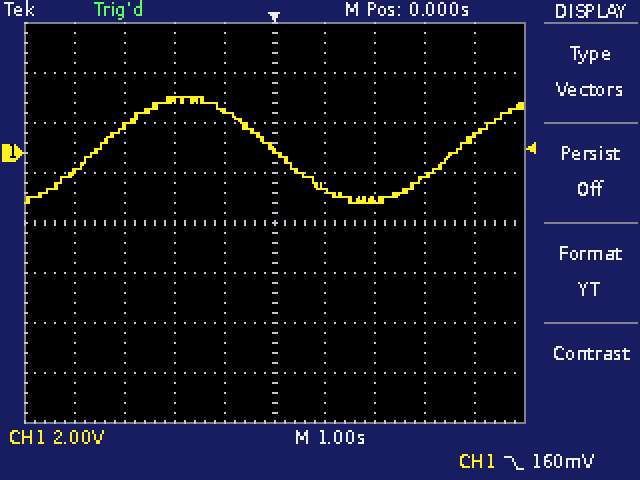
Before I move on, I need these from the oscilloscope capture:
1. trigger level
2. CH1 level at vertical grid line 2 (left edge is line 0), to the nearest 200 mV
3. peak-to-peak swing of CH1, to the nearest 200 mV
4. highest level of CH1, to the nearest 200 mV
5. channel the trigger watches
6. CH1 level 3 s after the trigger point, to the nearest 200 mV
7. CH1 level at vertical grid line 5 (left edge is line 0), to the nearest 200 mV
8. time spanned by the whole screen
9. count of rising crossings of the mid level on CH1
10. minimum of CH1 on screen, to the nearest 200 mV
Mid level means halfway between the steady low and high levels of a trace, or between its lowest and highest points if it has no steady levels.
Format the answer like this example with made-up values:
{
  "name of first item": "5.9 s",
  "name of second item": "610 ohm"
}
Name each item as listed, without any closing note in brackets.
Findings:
{
  "trigger level": "160 mV",
  "CH1 level at vertical grid line 2 (left edge is line 0), to the nearest 200 mV": "1.0 V",
  "peak-to-peak swing of CH1, to the nearest 200 mV": "4.2 V",
  "highest level of CH1, to the nearest 200 mV": "2.2 V",
  "channel the trigger watches": "CH1",
  "CH1 level 3 s after the trigger point, to the nearest 200 mV": "-1.0 V",
  "CH1 level at vertical grid line 5 (left edge is line 0), to the nearest 200 mV": "200 mV",
  "time spanned by the whole screen": "10 s",
  "count of rising crossings of the mid level on CH1": "2",
  "minimum of CH1 on screen, to the nearest 200 mV": "-2.0 V"
}
